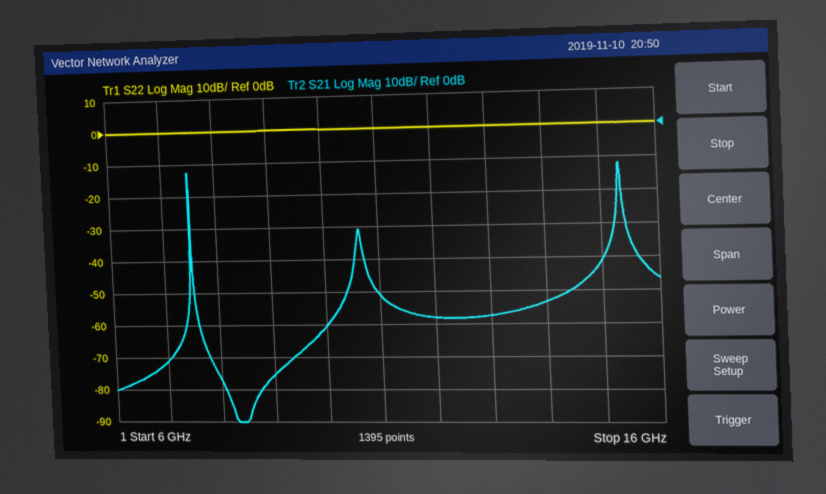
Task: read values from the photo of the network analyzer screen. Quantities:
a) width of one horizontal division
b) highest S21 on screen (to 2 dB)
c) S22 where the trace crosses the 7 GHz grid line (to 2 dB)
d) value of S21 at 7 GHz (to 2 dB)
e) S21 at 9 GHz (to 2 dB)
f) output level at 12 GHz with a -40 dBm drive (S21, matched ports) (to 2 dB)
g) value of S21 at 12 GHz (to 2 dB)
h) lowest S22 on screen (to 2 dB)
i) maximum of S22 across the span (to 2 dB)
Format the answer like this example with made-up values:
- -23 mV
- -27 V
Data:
- 1 GHz
- -12 dB
- 0 dB
- -72 dB
- -76 dB
- -98 dBm
- -58 dB
- 0 dB
- 0 dB
